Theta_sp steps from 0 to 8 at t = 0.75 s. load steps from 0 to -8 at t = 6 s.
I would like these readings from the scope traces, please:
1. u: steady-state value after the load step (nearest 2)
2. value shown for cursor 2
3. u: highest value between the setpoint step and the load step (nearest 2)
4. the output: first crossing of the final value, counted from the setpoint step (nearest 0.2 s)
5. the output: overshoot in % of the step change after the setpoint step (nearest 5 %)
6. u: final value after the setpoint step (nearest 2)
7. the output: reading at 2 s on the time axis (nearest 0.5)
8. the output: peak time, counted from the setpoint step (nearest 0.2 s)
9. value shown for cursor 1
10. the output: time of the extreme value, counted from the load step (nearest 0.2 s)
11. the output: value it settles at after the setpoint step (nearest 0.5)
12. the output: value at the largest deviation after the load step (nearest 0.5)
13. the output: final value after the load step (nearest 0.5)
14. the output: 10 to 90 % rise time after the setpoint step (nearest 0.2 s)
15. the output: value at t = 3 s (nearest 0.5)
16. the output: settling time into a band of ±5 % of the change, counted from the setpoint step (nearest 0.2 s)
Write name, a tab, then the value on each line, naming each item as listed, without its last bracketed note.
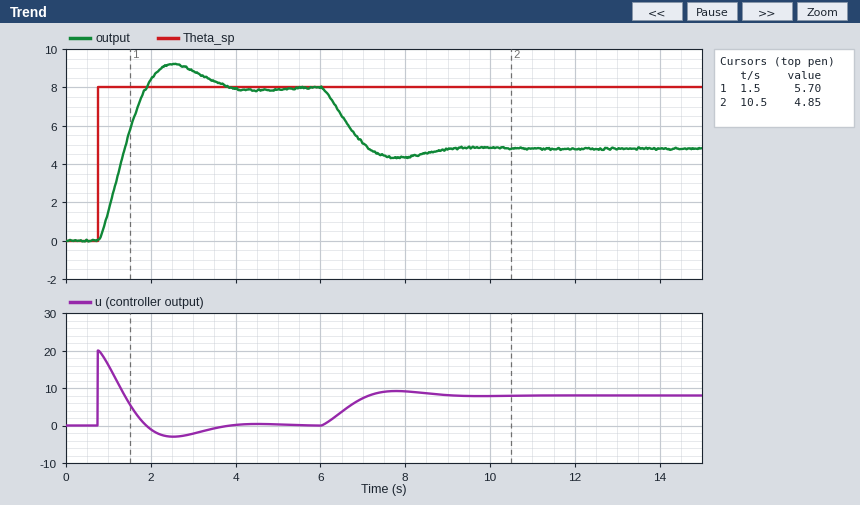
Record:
u: steady-state value after the load step	8
value shown for cursor 2	4.85
u: highest value between the setpoint step and the load step	20
the output: first crossing of the final value, counted from the setpoint step	1.2 s
the output: overshoot in % of the step change after the setpoint step	15 %
u: final value after the setpoint step	0
the output: reading at 2 s on the time axis	8.5
the output: peak time, counted from the setpoint step	1.8 s
value shown for cursor 1	5.70
the output: time of the extreme value, counted from the load step	1.8 s
the output: value it settles at after the setpoint step	8.0
the output: value at the largest deviation after the load step	4.5
the output: final value after the load step	5.0
the output: 10 to 90 % rise time after the setpoint step	0.8 s
the output: value at t = 3 s	9.0
the output: settling time into a band of ±5 % of the change, counted from the setpoint step	2.6 s
